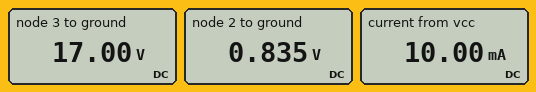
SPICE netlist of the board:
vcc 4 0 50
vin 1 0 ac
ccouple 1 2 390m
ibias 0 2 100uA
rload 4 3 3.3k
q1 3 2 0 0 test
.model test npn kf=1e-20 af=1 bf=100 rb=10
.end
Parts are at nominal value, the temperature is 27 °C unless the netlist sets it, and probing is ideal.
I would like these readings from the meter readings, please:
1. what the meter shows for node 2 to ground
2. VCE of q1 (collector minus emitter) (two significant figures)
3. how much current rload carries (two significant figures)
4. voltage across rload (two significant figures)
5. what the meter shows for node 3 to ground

0.835 V
17 V
10 mA
33 V
17.00 V
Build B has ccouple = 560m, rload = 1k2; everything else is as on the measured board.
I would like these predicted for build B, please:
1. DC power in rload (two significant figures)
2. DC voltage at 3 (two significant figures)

120 mW
38 V
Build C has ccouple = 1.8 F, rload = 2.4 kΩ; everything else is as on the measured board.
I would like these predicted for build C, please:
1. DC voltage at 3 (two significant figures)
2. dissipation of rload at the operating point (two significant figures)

26 V
240 mW
